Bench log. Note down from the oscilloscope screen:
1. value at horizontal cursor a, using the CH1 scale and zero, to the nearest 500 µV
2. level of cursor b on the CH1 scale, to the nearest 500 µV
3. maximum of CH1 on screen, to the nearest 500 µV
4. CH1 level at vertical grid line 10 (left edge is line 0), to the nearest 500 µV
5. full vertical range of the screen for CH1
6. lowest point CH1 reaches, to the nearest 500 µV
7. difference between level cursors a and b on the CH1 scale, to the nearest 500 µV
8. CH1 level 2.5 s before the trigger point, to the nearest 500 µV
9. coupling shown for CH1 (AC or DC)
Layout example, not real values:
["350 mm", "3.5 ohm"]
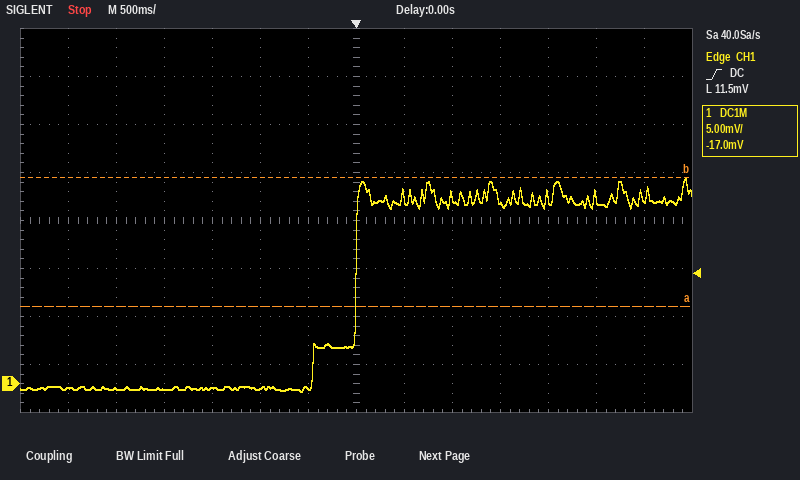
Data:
["8.0 mV", "21.5 mV", "21.5 mV", "19.0 mV", "40 mV", "-1.0 mV", "13.5 mV", "-500 µV", "DC"]
